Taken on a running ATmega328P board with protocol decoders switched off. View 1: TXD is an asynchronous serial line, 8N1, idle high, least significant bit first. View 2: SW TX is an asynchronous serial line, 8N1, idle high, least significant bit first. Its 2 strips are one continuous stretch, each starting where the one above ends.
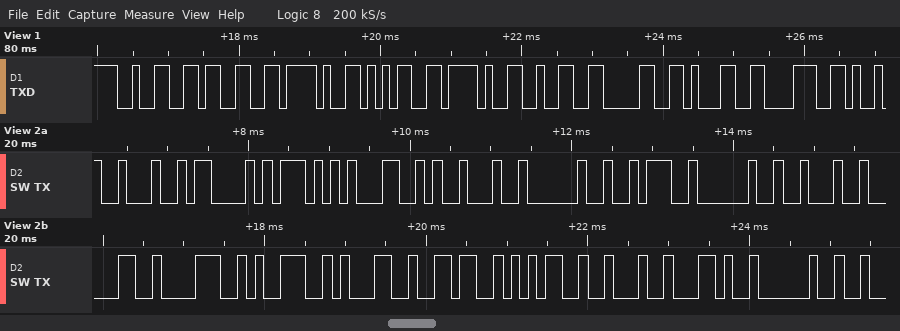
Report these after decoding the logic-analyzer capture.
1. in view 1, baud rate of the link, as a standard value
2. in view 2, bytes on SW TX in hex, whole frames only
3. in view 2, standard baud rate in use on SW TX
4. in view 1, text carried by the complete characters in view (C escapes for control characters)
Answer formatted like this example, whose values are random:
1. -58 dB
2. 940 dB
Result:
1. 9600 baud
2. 22 43 57 4C 22 20 3A 20 22 30 38 39 31 36 35 22 2C 20
3. 9600 baud
4. "23/5/2018"
